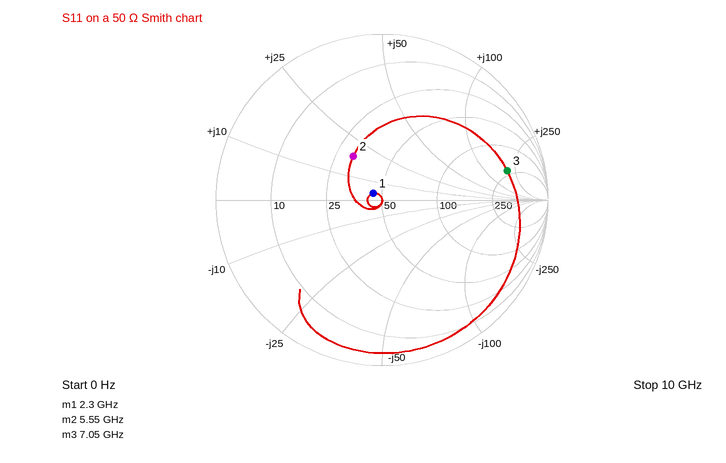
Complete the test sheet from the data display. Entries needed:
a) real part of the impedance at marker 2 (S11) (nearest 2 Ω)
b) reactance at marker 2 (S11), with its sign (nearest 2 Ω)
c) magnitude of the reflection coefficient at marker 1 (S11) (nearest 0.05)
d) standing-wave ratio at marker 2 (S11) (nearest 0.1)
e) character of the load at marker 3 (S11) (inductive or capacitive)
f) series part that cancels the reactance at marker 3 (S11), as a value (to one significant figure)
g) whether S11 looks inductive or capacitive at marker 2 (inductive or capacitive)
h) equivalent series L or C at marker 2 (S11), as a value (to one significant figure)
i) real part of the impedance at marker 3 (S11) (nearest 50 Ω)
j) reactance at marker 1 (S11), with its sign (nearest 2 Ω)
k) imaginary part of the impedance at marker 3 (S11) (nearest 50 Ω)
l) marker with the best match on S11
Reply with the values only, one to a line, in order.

32 Ω
+18 Ω
0.05
1.9
inductive
100 fF
inductive
500 pH
200 Ω
+4 Ω
+200 Ω
marker 1
